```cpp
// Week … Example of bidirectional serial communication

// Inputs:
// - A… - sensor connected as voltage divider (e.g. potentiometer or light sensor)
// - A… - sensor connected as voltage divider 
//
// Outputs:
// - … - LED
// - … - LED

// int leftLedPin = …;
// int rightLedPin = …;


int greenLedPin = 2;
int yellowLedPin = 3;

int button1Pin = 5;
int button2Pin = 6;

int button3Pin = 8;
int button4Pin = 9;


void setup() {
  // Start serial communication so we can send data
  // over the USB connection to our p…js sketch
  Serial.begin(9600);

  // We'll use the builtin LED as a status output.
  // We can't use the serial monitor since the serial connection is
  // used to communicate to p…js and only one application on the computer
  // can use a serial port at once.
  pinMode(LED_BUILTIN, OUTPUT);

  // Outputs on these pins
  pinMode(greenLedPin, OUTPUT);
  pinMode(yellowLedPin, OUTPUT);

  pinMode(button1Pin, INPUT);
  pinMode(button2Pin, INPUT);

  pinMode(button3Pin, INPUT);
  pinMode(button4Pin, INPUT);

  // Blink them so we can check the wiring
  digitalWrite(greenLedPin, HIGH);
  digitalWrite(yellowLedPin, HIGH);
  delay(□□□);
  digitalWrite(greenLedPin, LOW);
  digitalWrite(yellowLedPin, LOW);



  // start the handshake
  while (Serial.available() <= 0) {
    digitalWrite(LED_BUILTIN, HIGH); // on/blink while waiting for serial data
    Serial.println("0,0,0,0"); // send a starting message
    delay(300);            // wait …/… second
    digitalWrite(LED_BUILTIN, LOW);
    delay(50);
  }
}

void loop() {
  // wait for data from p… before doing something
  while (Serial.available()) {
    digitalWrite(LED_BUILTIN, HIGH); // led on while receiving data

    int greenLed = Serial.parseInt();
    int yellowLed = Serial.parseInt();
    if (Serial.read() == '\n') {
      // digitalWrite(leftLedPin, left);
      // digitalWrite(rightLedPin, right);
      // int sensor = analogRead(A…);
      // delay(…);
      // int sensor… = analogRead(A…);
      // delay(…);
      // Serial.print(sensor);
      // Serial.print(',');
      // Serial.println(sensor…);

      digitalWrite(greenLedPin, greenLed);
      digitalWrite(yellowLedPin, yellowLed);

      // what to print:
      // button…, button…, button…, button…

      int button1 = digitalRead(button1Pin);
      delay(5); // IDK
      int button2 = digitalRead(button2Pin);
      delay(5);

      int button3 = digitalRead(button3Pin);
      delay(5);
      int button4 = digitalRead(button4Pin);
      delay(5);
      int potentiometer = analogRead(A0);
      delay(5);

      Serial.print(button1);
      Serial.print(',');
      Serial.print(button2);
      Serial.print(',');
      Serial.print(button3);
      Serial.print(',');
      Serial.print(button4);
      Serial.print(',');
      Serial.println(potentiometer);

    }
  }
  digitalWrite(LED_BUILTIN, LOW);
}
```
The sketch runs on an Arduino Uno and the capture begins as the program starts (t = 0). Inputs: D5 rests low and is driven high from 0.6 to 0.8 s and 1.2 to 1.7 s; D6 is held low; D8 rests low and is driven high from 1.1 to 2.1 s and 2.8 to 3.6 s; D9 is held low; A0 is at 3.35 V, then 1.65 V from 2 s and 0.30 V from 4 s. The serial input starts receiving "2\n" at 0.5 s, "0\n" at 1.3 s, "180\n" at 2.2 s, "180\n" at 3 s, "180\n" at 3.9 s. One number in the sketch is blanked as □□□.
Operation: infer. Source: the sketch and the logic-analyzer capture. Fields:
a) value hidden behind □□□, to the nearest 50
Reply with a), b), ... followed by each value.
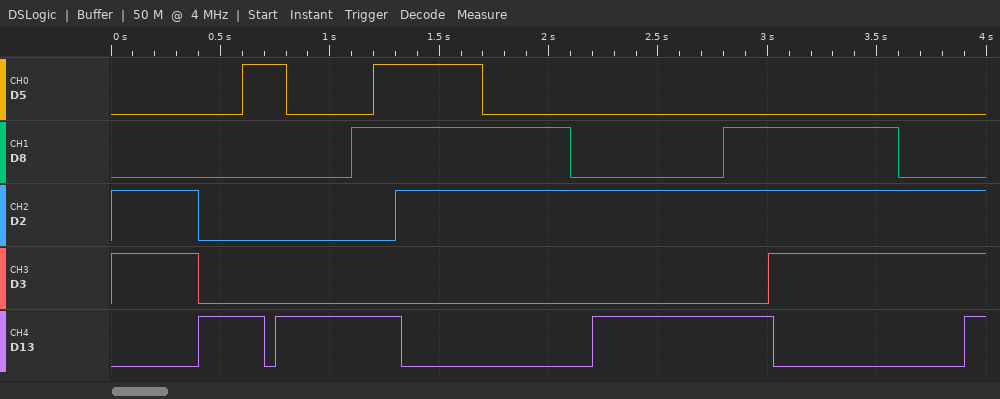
a) 400
